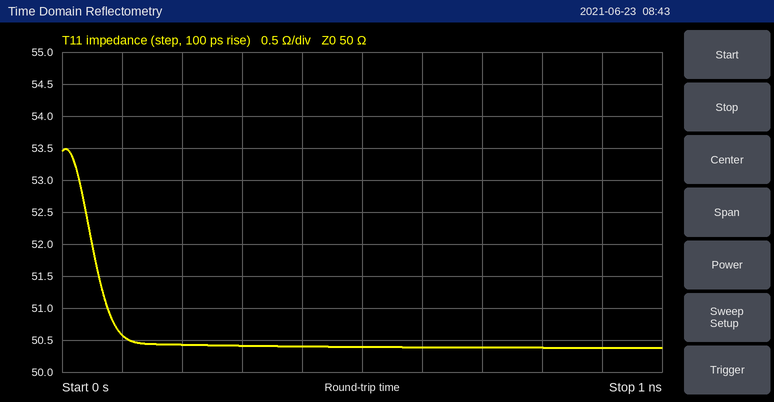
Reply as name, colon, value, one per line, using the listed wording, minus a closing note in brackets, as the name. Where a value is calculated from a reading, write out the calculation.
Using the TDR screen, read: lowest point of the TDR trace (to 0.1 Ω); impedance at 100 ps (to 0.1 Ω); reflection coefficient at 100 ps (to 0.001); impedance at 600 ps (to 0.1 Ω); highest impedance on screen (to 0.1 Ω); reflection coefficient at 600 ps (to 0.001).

lowest point of the TDR trace: 50.4 Ω
impedance at 100 ps: 50.6 Ω
reflection coefficient at 100 ps: (50.6 − 50)/(50.6 + 50) ≈ +0.006
impedance at 600 ps: 50.4 Ω
highest impedance on screen: 53.5 Ω
reflection coefficient at 600 ps: (50.4 − 50)/(50.4 + 50) ≈ +0.004
